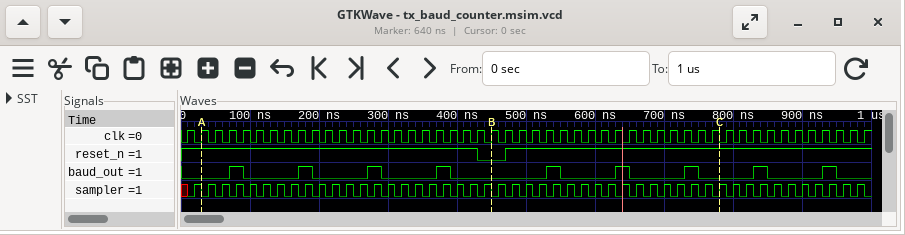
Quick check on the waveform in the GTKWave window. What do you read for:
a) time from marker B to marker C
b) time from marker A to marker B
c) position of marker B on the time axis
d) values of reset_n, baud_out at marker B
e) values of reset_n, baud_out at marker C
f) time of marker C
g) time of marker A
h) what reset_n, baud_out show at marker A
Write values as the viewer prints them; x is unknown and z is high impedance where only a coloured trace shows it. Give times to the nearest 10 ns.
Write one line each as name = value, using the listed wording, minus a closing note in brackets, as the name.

time from marker B to marker C = 330 ns
time from marker A to marker B = 420 ns
position of marker B on the time axis = 450 ns
values of reset_n, baud_out at marker B = reset_n=0, baud_out=0
values of reset_n, baud_out at marker C = reset_n=1, baud_out=0
time of marker C = 780 ns
time of marker A = 30 ns
what reset_n, baud_out show at marker A = reset_n=1, baud_out=0
